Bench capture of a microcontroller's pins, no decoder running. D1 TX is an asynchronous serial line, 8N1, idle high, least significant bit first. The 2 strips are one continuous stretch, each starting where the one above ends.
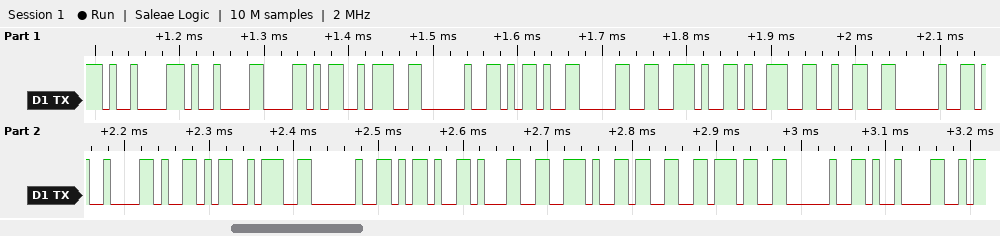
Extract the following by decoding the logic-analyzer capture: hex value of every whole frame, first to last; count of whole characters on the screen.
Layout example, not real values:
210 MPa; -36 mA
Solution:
09 09 58 3A 20 2D 30 2E 39 32 20 09 59 3A 20 2D 31 2E 33 37 20 09; 22
